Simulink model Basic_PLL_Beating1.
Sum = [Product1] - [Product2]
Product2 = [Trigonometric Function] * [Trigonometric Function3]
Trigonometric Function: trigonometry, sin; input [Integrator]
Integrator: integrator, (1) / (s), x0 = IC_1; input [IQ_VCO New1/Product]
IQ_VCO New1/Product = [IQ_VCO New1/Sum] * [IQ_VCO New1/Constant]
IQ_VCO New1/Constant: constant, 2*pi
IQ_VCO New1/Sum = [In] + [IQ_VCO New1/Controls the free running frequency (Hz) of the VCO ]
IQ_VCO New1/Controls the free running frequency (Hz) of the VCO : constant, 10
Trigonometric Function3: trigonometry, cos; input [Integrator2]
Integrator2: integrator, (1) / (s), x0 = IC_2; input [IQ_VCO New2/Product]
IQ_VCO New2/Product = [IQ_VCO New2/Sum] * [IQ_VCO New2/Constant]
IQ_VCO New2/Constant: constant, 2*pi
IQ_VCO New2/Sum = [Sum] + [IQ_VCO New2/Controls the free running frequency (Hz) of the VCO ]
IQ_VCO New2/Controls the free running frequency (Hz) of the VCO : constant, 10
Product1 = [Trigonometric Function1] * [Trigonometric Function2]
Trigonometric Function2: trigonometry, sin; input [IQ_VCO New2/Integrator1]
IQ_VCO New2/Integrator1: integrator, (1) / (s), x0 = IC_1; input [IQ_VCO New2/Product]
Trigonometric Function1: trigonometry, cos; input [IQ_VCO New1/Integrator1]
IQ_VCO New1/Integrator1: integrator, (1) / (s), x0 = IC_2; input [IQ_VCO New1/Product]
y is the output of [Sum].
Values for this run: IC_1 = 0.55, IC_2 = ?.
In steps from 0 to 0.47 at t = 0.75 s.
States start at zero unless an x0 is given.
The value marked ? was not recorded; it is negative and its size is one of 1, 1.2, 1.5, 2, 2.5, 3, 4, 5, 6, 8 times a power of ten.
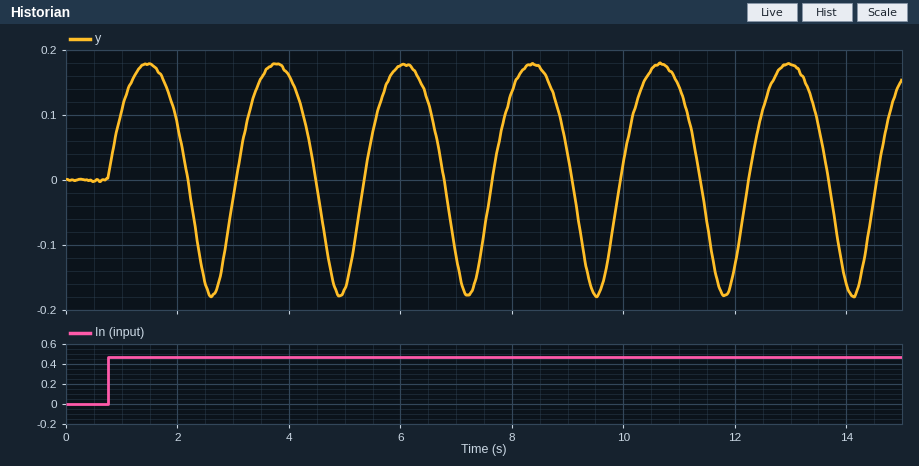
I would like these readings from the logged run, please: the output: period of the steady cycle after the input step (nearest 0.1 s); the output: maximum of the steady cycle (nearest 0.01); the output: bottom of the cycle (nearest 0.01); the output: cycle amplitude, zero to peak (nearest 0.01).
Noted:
2.3 s
0.18
-0.18
0.18
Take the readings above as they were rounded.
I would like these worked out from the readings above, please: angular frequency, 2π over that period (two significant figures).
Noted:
2.7 rad/s
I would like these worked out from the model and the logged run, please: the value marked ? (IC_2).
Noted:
-1.2
